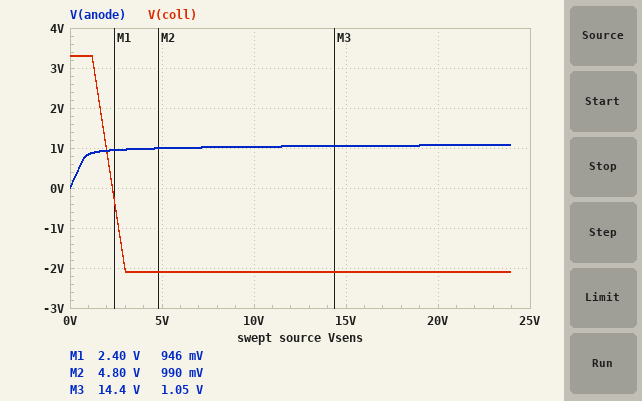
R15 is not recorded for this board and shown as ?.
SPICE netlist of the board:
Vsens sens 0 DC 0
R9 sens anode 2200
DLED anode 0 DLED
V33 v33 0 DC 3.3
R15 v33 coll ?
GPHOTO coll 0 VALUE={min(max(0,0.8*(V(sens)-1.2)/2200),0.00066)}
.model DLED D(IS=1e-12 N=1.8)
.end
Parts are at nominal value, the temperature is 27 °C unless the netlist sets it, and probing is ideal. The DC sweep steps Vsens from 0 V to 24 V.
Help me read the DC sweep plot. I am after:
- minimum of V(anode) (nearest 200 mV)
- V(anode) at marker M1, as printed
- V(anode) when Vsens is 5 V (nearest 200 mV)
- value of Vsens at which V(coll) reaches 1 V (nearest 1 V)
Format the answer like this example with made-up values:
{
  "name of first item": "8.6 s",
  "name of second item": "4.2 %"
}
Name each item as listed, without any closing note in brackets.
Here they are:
{
  "minimum of V(anode)": "0 V",
  "V(anode) at marker M1, as printed": "946 mV",
  "V(anode) when Vsens is 5 V": "1.0 V",
  "value of Vsens at which V(coll) reaches 1 V": "2 V"
}
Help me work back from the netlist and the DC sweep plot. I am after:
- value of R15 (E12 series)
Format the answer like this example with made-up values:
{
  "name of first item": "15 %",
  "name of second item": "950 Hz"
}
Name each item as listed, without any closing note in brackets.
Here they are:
{
  "value of R15": "8.2 kΩ"
}
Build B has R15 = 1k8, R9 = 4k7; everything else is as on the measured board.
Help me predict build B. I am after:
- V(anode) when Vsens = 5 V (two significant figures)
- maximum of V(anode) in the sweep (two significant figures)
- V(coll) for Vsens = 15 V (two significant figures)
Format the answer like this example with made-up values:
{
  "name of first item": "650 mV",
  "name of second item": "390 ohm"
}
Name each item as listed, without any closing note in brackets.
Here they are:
{
  "V(anode) when Vsens = 5 V": "960 mV",
  "maximum of V(anode) in the sweep": "1.0 V",
  "V(coll) for Vsens = 15 V": "2.1 V"
}
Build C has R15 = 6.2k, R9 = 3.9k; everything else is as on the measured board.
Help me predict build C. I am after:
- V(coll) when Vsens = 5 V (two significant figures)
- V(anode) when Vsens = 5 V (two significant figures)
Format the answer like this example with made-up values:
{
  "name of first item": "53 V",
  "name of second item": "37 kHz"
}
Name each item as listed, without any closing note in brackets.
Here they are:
{
  "V(coll) when Vsens = 5 V": "-790 mV",
  "V(anode) when Vsens = 5 V": "970 mV"
}
